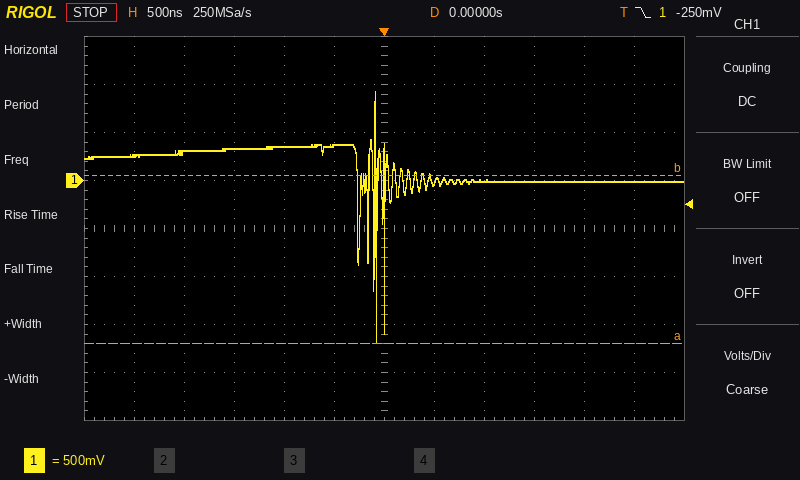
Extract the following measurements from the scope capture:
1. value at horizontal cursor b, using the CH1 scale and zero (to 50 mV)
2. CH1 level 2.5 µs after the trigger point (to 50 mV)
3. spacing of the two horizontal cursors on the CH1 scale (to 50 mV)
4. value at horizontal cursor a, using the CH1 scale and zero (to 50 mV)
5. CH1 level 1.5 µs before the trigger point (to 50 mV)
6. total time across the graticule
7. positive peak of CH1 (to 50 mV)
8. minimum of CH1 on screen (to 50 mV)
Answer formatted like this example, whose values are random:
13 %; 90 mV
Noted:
50 mV; 0 mV; 1.75 V; -1.70 V; 350 mV; 6 µs; 950 mV; -1.70 V
